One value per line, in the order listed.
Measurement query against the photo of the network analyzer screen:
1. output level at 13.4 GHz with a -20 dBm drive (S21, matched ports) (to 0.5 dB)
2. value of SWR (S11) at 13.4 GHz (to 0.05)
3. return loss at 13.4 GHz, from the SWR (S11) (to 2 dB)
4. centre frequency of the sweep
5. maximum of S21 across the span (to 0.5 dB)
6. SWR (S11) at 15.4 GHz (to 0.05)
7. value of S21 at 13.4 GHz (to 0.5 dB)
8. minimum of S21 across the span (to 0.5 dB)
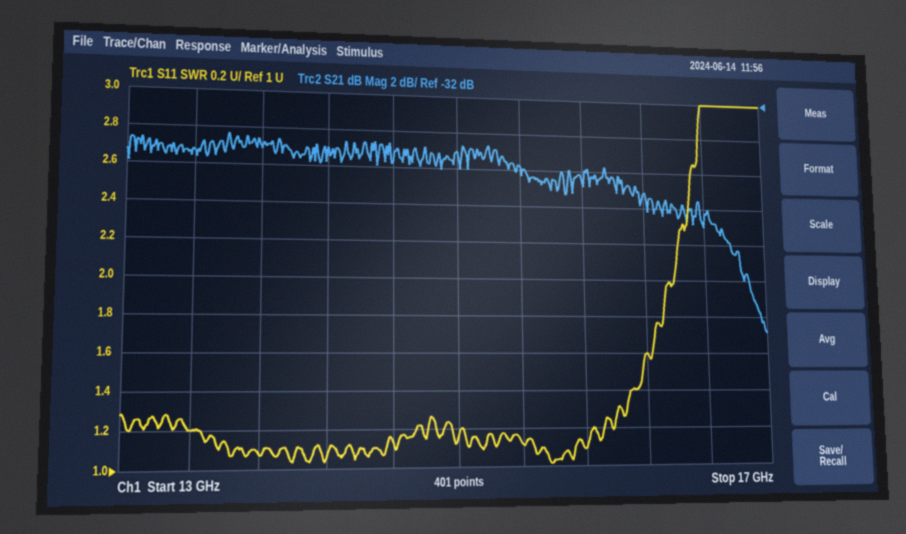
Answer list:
-55.5 dBm
1.20
20 dB
15 GHz
-34.5 dB
1.10
-35.5 dB
-45.0 dB
